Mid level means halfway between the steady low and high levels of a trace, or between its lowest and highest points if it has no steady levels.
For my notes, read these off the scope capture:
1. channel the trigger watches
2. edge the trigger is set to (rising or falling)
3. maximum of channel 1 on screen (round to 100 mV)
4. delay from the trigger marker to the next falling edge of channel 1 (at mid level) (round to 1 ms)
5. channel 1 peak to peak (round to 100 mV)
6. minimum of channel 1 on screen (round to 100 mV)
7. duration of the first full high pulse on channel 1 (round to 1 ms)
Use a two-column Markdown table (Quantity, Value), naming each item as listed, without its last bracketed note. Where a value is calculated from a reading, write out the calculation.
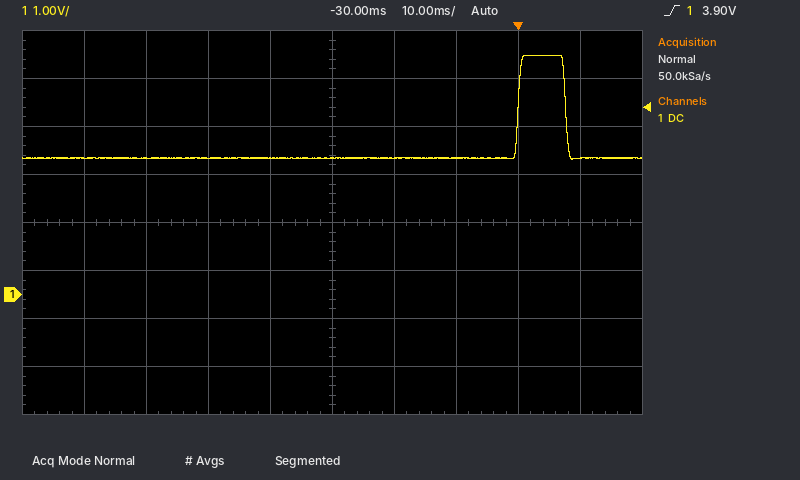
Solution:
| Quantity | Value |
|---|---|
| channel the trigger watches | channel 1 |
| edge the trigger is set to | rising |
| maximum of channel 1 on screen | 5.0 V |
| delay from the trigger marker to the next falling edge of channel 1 (at mid level) | 8 ms |
| channel 1 peak to peak | 5.0 V − (2.8 V) = 2.2 V |
| minimum of channel 1 on screen | 2.8 V |
| duration of the first full high pulse on channel 1 | 8 ms |
